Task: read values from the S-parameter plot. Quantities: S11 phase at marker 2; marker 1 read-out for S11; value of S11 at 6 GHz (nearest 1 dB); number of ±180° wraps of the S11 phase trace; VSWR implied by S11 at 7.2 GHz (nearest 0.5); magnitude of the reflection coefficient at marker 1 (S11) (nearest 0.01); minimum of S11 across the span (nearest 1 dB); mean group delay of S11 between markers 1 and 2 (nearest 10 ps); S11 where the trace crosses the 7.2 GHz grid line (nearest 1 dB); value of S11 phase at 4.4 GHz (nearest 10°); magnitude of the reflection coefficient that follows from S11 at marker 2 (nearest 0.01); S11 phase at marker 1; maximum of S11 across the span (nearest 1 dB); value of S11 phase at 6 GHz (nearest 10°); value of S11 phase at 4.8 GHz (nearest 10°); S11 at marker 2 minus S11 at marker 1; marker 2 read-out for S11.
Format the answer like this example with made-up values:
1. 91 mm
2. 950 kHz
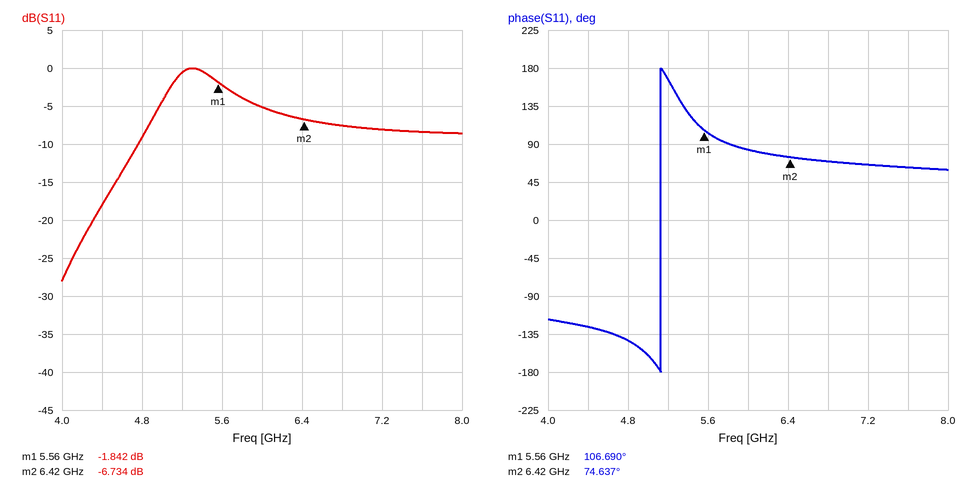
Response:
1. 74.637°
2. -1.842 dB
3. -5 dB
4. 1
5. 2.5
6. 0.81
7. -28 dB
8. 100 ps
9. -8 dB
10. -130°
11. 0.46
12. 106.690°
13. 0 dB
14. 80°
15. -140°
16. -4.892 dB
17. -6.734 dB
